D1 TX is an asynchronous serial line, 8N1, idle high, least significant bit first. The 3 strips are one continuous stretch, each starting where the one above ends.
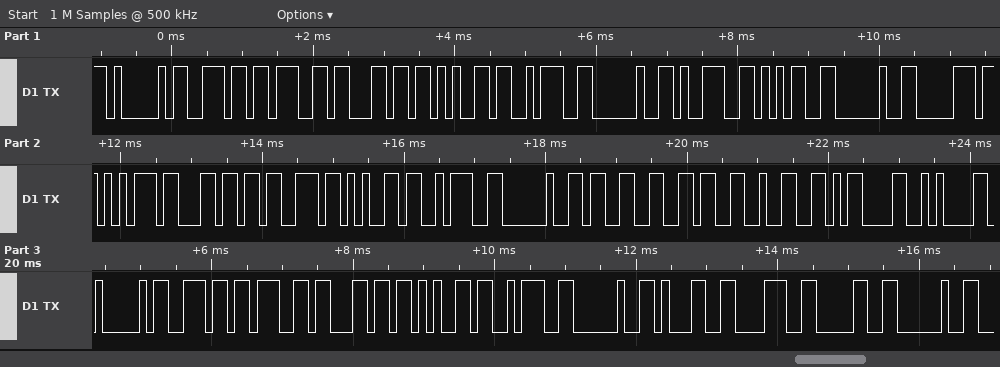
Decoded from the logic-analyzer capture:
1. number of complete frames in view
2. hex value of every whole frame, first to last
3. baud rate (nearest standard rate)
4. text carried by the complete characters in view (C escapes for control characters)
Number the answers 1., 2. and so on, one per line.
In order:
1. 33
2. 41 6E 67 6C 65 3A 20 39 35 20 70 75 6C 73 65 3A 20 33 36 32 0D 0A 41 6E 67 6C 65 3A 20 31 38 30 20
3. 9600 baud
4. "Angle: 95 pulse: 362\r\nAngle: 180 "
